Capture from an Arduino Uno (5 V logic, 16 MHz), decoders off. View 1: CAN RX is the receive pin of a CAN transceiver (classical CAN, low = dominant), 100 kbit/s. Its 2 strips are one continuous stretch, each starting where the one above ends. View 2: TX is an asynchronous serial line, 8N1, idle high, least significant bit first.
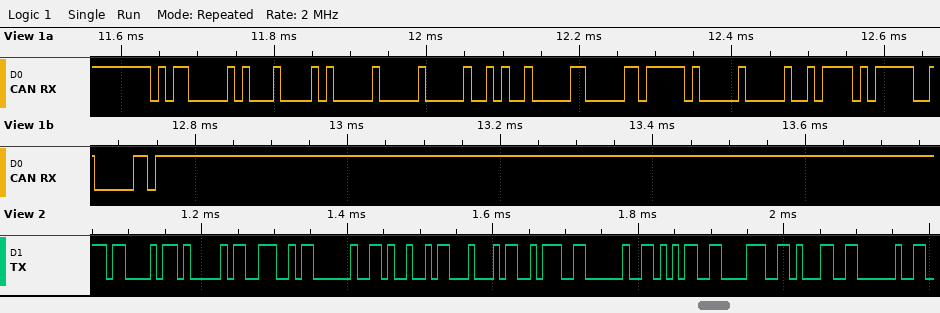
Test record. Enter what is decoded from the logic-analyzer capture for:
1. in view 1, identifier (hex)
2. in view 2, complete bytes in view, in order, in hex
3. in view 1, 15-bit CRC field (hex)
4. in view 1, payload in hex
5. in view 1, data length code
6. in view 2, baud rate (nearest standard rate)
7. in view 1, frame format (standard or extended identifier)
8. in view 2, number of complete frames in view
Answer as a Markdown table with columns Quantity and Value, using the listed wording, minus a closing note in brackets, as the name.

| Quantity | Value |
|---|---|
| in view 1, identifier | 0x581 |
| in view 2, complete bytes in view, in order, in hex | 43 41 4E 20 49 44 3A 20 35 38 31 20 |
| in view 1, 15-bit CRC field | 0x2FA0 |
| in view 1, payload in hex | 50 00 05 20 82 FC 00 2F |
| in view 1, data length code | 8 |
| in view 2, baud rate | 115200 baud |
| in view 1, frame format | standard |
| in view 2, number of complete frames in view | 12 |
